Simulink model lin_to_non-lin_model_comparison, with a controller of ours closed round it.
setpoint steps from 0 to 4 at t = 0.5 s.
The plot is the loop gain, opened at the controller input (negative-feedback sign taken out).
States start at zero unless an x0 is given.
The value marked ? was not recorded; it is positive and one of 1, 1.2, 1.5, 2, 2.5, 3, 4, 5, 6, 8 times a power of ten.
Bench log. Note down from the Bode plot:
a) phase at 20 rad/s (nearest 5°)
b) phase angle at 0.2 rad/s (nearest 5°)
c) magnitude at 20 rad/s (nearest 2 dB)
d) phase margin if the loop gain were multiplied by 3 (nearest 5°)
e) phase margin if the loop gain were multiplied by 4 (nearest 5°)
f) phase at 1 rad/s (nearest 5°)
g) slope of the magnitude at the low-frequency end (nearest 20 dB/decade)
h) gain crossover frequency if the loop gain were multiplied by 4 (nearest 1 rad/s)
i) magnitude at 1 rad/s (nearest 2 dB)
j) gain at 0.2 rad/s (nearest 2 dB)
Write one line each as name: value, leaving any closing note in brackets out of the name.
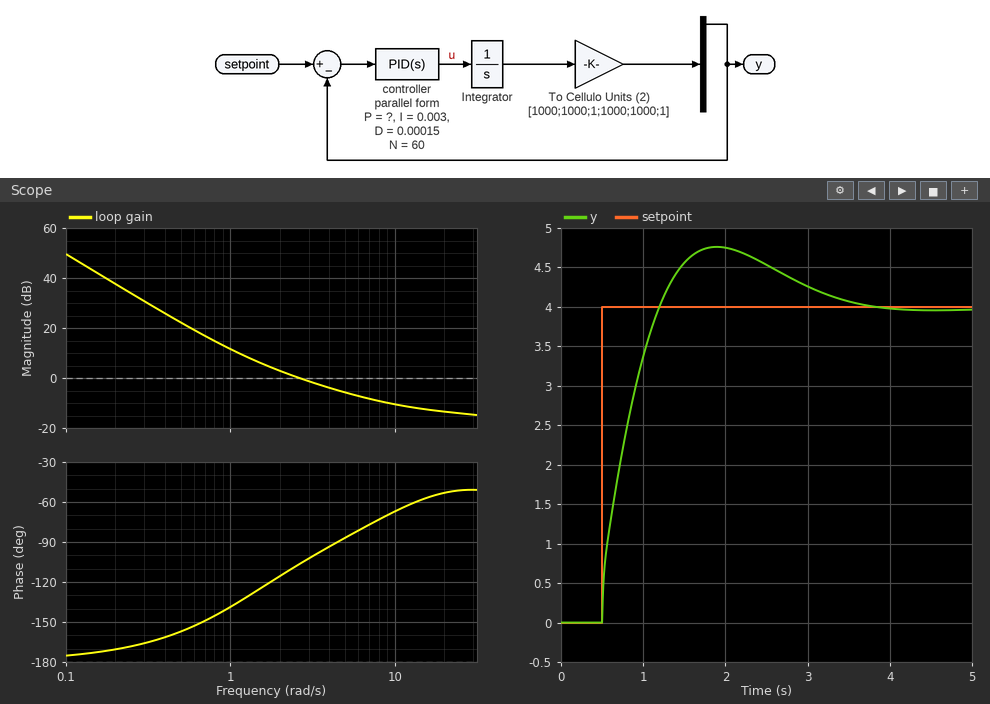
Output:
phase at 20 rad/s: -55°
phase angle at 0.2 rad/s: -170°
magnitude at 20 rad/s: -14 dB
phase margin if the loop gain were multiplied by 3: 110°
phase margin if the loop gain were multiplied by 4: 120°
phase at 1 rad/s: -140°
slope of the magnitude at the low-frequency end: -40 dB/decade
gain crossover frequency if the loop gain were multiplied by 4: 14 rad/s
magnitude at 1 rad/s: 12 dB
gain at 0.2 rad/s: 38 dB
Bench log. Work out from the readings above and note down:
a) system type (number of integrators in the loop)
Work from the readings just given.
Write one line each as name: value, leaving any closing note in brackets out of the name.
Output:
system type: 2
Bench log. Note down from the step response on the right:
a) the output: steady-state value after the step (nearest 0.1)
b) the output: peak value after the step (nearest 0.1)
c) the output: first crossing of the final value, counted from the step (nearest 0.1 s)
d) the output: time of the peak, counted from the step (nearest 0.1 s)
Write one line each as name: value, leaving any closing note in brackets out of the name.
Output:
the output: steady-state value after the step: 4.0
the output: peak value after the step: 4.8
the output: first crossing of the final value, counted from the step: 0.7 s
the output: time of the peak, counted from the step: 1.4 s
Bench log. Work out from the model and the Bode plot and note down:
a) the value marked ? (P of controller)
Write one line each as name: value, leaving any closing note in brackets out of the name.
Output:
the value marked ?: 0.0025
